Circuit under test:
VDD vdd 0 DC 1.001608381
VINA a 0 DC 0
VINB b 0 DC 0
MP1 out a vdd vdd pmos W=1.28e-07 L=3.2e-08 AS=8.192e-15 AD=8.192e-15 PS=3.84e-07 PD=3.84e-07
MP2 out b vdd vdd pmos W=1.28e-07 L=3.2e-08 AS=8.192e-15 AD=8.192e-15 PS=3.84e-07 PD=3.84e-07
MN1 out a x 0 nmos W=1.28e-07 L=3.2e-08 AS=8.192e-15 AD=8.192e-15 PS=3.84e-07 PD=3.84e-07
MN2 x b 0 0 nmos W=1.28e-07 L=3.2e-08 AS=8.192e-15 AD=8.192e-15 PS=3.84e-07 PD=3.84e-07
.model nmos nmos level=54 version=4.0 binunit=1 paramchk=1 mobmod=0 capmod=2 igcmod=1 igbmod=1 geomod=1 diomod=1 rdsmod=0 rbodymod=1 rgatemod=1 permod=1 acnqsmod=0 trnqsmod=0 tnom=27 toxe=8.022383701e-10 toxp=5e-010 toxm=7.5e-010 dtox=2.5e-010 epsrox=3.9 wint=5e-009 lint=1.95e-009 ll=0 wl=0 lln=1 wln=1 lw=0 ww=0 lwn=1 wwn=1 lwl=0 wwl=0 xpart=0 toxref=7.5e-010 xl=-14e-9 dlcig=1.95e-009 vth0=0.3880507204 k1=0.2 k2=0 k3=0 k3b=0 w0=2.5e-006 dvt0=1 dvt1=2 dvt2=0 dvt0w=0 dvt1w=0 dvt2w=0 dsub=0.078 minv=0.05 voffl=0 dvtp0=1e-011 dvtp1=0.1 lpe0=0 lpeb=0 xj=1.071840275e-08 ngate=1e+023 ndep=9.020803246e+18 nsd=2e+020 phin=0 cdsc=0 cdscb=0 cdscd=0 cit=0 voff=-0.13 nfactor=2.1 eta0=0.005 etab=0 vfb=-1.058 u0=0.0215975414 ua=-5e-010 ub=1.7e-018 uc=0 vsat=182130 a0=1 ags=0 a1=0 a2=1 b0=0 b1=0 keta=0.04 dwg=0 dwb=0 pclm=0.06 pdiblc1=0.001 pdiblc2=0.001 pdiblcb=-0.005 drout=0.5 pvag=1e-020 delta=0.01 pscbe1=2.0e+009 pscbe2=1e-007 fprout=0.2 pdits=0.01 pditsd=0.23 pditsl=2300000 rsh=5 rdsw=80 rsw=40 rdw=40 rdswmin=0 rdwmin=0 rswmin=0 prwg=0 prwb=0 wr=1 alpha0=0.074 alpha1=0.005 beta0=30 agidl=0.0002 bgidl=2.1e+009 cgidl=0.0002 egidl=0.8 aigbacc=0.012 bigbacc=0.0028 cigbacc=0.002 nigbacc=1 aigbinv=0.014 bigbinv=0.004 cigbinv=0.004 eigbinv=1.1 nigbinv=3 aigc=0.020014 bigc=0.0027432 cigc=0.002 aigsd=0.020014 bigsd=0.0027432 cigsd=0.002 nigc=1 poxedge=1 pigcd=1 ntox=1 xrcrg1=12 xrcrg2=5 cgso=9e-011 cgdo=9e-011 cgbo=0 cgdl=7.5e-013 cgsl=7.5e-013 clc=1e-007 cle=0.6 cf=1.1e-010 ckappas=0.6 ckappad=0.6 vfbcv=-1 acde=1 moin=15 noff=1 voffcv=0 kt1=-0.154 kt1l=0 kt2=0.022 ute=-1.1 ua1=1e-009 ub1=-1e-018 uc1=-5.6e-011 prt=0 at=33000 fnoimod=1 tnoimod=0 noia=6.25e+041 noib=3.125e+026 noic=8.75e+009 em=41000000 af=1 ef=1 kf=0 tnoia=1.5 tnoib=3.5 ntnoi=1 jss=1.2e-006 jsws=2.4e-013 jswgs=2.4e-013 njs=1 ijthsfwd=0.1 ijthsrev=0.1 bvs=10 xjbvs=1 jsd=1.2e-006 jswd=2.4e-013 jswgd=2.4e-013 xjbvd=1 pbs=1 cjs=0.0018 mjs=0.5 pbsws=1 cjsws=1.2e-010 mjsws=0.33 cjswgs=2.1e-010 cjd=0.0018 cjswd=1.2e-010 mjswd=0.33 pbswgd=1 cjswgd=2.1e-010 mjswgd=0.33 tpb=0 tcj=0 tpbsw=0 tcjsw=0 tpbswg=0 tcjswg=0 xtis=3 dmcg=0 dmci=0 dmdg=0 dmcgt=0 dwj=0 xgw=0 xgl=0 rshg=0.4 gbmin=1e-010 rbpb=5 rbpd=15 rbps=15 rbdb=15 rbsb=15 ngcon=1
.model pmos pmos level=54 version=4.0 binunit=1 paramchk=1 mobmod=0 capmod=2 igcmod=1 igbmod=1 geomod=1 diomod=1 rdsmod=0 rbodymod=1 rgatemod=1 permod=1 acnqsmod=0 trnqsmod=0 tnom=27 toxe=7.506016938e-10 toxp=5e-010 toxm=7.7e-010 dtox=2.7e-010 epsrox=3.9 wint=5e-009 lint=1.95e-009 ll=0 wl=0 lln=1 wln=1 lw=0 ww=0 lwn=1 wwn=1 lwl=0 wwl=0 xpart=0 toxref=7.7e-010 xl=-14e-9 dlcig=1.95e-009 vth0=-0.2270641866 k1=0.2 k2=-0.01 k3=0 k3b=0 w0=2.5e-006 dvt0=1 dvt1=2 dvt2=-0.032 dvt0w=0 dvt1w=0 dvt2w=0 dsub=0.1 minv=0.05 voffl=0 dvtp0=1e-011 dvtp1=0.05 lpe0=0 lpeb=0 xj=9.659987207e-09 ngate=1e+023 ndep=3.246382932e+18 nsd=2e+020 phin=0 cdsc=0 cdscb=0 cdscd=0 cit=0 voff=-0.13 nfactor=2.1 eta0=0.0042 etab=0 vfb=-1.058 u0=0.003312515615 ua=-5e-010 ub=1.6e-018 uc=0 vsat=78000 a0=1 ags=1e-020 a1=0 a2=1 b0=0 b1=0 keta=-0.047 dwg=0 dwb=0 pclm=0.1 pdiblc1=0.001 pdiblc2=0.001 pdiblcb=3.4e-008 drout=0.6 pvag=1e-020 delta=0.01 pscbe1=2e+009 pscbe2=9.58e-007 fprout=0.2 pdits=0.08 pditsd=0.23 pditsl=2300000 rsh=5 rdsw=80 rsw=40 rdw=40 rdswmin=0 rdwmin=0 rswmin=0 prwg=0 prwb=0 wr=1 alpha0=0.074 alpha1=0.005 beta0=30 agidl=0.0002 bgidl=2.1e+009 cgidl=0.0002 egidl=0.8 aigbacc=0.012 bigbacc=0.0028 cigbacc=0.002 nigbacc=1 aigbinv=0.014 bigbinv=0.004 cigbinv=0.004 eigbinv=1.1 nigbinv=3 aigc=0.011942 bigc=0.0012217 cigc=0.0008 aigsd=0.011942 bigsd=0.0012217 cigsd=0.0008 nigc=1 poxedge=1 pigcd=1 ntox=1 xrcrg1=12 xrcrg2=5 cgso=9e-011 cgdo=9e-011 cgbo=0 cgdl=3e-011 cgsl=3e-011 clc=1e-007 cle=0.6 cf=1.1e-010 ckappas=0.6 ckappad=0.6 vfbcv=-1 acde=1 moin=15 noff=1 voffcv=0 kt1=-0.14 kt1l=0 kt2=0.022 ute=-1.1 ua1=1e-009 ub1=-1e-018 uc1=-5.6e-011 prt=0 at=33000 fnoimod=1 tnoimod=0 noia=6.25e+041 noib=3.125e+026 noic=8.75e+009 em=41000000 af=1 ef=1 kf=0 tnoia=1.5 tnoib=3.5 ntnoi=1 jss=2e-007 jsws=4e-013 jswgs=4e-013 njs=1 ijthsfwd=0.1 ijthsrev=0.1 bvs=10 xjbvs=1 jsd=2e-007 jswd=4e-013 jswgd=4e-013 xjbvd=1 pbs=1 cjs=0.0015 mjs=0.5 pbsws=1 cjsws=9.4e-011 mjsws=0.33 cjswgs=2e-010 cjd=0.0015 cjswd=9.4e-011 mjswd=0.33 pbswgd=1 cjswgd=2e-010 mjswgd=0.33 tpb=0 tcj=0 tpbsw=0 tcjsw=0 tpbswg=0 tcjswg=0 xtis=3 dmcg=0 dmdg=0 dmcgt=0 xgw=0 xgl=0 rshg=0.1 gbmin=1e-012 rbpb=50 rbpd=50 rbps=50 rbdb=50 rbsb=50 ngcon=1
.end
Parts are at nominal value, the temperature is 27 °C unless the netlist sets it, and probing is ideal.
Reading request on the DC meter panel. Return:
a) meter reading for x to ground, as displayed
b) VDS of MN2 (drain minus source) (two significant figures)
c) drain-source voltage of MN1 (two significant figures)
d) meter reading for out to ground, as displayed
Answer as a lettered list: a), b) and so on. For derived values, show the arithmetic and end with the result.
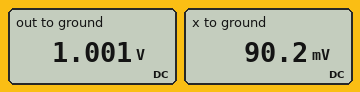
a) 90.2 mV
b) 90.2 mV = 90 mV
c) 1.001 V - 90.2 mV = 910 mV
d) 1.001 V
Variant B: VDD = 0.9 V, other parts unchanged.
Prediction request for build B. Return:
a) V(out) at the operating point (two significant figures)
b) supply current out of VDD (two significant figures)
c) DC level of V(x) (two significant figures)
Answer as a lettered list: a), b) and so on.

a) 900 mV
b) 120 nA
c) 81 mV
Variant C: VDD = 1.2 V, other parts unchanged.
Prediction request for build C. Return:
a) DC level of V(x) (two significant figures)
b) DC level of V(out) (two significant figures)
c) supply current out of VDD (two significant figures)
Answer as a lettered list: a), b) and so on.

a) 110 mV
b) 1.2 V
c) 580 nA
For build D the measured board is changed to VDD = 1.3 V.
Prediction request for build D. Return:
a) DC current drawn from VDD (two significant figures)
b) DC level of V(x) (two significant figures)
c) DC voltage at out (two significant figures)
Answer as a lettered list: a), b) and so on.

a) 1.3 µA
b) 120 mV
c) 1.3 V
